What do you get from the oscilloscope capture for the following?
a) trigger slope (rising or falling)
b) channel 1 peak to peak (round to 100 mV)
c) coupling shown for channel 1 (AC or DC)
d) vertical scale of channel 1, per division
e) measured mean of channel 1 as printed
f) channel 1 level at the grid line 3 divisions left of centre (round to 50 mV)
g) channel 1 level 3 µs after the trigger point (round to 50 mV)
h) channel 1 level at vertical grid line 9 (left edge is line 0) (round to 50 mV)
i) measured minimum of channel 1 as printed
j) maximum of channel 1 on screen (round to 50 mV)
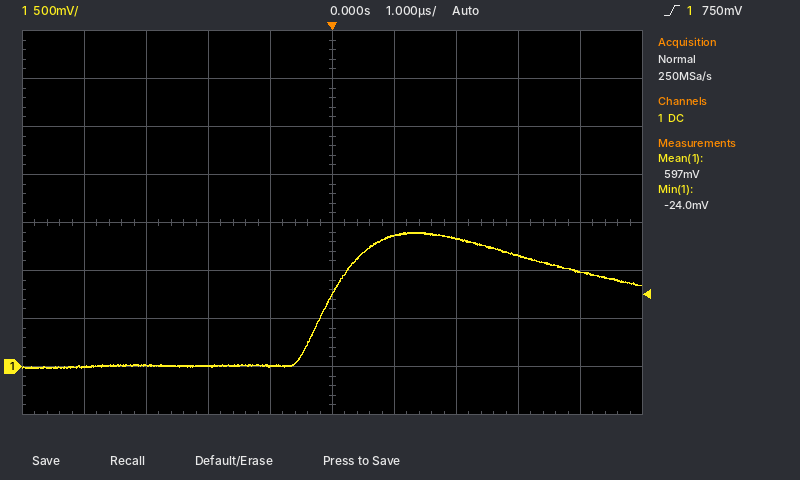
rising
1.40 V
DC
500 mV
597 mV
0 mV
1.15 V
1.00 V
-24.0 mV
1.40 V
